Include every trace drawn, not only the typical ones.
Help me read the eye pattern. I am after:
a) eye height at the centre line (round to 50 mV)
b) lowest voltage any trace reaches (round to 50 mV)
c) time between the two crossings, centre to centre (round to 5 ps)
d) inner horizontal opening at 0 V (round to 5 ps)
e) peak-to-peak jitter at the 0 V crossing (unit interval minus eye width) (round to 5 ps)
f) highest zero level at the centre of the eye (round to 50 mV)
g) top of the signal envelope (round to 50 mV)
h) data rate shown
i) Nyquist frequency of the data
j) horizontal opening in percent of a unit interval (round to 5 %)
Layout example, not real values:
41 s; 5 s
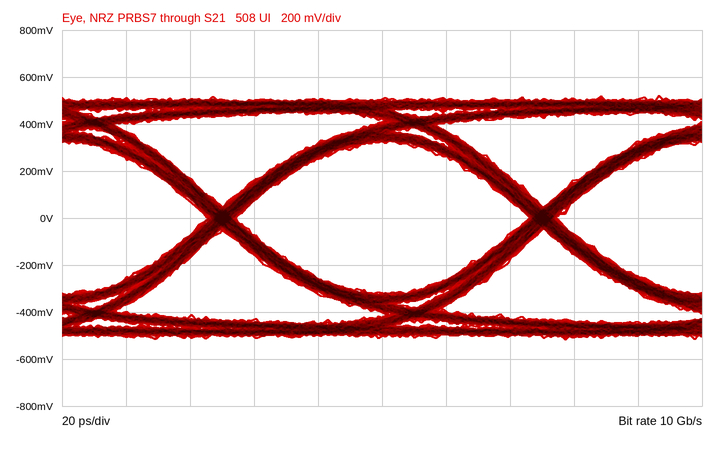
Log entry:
650 mV; -500 mV; 100 ps; 90 ps; 10 ps; -300 mV; 500 mV; 10 Gb/s; 5 GHz; 90 %
